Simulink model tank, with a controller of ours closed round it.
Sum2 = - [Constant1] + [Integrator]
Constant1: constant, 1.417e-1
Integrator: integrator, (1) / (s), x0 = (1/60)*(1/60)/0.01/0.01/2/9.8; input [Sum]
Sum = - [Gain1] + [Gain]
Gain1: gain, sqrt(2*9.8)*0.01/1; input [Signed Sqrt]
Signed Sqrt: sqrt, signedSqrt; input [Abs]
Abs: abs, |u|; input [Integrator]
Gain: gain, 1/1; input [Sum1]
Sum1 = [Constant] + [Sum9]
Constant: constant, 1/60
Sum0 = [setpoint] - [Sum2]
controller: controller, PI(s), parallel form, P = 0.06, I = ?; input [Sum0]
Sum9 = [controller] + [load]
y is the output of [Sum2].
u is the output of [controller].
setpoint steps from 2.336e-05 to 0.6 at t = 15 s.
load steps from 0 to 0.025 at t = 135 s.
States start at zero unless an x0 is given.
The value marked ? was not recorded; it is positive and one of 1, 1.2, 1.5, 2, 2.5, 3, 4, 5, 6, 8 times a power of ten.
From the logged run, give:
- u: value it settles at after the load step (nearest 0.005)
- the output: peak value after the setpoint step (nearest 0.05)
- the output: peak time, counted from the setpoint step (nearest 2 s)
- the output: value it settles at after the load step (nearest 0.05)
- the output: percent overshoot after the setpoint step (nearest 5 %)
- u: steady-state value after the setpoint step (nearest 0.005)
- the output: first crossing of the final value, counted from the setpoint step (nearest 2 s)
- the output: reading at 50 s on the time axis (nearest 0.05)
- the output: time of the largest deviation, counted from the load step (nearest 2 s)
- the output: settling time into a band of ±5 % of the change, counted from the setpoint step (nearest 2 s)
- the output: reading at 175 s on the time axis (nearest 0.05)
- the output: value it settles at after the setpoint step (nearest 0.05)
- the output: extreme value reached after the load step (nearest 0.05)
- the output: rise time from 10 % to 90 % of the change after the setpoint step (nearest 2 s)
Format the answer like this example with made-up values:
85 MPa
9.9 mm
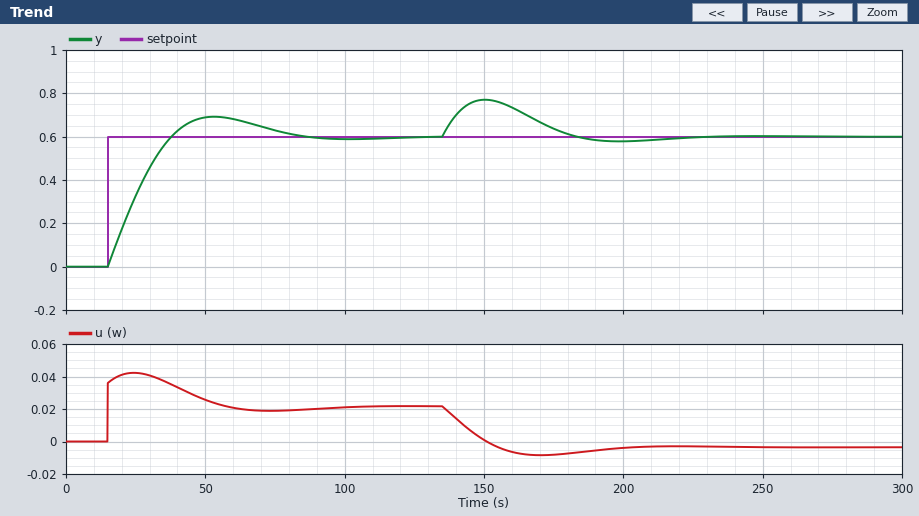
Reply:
-0.005
0.70
38 s
0.60
15 %
0.020
22 s
0.70
16 s
60 s
0.65
0.60
0.75
18 s
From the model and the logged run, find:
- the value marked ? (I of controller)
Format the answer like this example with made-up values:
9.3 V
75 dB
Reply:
0.006
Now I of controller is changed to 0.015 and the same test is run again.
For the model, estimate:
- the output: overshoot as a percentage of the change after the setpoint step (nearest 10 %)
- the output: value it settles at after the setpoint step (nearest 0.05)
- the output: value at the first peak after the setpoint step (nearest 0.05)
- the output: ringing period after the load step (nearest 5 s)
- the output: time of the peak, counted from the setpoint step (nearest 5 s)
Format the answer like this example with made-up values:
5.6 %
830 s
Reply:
30 %
0.60
0.80
55 s
25 s
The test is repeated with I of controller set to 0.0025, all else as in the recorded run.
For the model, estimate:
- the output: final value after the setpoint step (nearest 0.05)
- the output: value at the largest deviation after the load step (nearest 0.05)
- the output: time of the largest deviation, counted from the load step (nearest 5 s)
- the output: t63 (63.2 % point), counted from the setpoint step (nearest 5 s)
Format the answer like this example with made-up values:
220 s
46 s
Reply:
0.60
0.80
20 s
15 s
